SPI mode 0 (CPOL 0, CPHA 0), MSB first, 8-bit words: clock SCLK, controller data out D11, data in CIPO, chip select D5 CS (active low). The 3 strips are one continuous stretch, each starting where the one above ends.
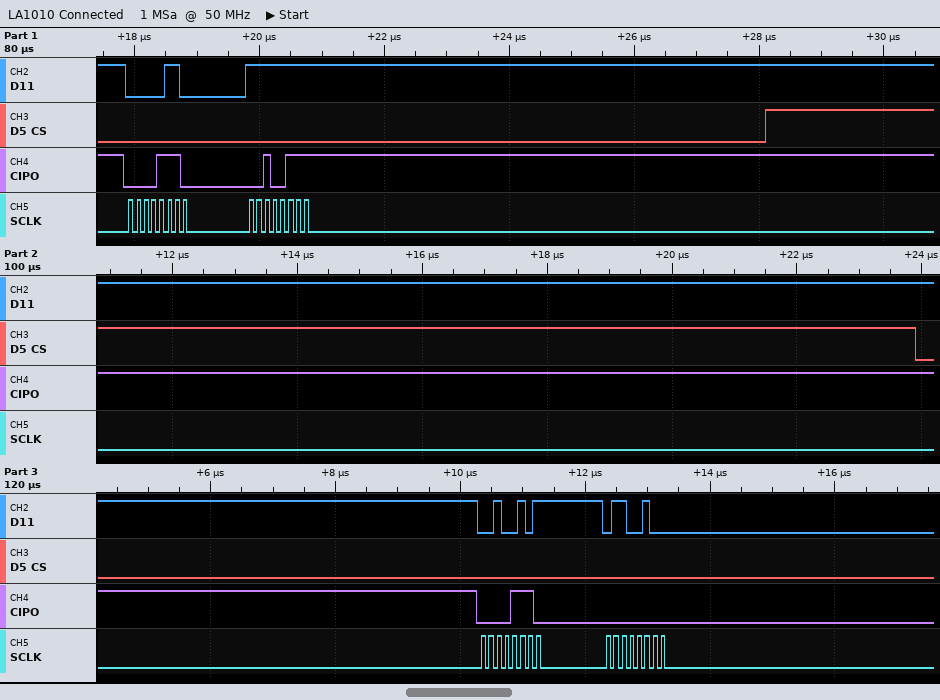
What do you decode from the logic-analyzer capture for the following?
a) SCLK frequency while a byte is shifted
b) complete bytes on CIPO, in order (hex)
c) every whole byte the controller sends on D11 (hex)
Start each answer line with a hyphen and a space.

- 8 MHz
- 0x0E 0x27 0x0E 0x00
- 0x06 0xFF 0x25 0x64
